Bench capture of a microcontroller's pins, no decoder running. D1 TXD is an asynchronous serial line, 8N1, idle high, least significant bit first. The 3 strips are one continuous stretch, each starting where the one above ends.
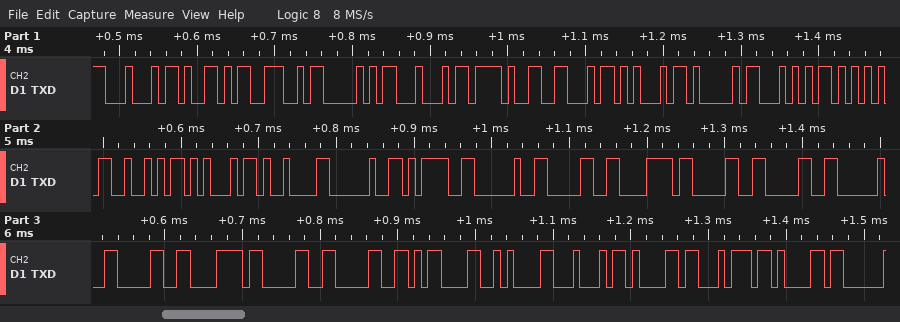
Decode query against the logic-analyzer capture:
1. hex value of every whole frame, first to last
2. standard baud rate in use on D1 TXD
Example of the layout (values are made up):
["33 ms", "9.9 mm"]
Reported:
["44 59 4E 50 44 2F 46 45 41 54 55 52 45 09 20 3D 20 30 78 30 30 20 30 78 30 30 0D 0A 44 61 74 61", "115200 baud"]
